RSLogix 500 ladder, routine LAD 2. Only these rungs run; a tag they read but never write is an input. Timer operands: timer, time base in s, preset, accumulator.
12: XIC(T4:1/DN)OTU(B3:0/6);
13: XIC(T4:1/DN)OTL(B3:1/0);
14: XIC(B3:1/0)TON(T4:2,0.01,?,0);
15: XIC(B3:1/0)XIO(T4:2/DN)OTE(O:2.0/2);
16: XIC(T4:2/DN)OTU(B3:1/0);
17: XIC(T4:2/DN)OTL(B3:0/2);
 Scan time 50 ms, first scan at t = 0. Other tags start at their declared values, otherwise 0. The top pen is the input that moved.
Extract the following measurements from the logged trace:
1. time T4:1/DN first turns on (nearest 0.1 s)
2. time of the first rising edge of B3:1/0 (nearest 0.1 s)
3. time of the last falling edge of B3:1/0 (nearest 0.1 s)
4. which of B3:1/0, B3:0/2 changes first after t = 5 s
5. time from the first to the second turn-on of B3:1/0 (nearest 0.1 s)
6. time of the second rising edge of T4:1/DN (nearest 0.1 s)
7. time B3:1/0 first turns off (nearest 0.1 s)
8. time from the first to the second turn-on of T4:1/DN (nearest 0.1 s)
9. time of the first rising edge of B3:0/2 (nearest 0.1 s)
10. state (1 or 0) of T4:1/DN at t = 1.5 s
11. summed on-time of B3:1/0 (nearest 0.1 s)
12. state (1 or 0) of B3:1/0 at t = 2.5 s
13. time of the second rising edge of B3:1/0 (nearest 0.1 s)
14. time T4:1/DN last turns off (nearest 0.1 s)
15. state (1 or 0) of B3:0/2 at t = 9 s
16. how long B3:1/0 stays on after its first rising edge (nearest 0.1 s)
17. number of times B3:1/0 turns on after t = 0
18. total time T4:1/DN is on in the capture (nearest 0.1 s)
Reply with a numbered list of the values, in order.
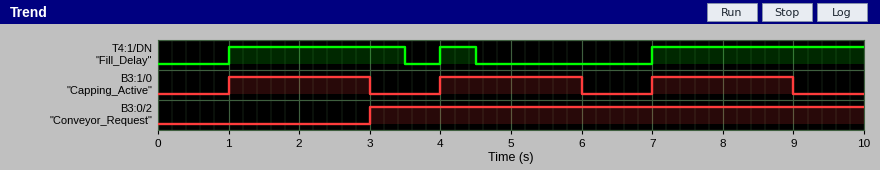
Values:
1. 1.0 s
2. 1.0 s
3. 9.0 s
4. B3:1/0
5. 3.0 s
6. 4.0 s
7. 3.0 s
8. 3.0 s
9. 3.0 s
10. 1
11. 6.0 s
12. 1
13. 4.0 s
14. 4.5 s
15. 1
16. 2.0 s
17. 3
18. 6.0 s
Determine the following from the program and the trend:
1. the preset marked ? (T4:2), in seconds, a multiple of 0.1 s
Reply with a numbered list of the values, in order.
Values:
1. 2.0 s
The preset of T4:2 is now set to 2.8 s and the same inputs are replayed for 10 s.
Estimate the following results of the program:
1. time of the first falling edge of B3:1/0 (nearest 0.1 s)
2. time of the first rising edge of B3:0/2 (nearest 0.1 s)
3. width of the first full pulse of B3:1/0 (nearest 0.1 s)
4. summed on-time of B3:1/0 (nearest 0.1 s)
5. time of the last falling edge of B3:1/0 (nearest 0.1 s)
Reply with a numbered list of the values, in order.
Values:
1. 3.8 s
2. 3.8 s
3. 2.8 s
4. 8.4 s
5. 9.8 s
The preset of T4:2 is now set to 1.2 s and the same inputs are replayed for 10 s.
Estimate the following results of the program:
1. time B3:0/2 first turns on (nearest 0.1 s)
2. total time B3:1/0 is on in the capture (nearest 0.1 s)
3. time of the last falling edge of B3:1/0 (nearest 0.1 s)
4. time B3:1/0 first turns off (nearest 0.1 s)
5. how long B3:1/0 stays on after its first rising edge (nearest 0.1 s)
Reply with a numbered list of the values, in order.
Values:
1. 2.2 s
2. 3.6 s
3. 8.2 s
4. 2.2 s
5. 1.2 s
